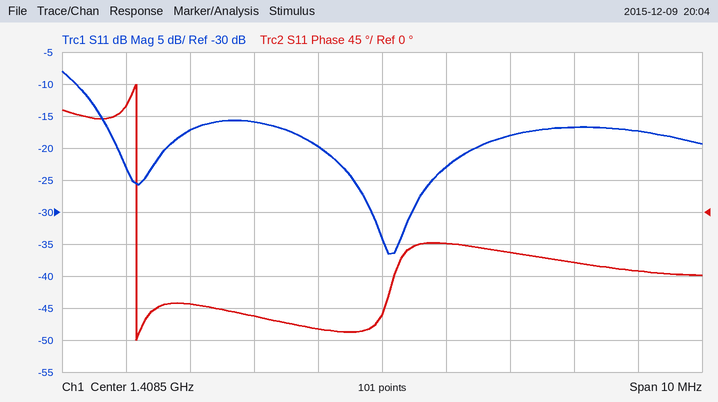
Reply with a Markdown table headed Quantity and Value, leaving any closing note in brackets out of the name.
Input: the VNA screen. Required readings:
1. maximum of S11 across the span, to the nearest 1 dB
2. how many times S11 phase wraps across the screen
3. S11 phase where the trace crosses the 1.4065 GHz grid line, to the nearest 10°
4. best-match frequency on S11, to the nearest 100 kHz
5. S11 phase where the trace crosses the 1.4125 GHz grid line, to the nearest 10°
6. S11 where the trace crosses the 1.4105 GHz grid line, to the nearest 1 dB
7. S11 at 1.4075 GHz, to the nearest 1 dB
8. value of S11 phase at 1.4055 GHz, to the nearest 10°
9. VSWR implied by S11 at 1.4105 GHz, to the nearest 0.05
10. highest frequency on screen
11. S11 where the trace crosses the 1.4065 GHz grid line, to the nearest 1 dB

| Quantity | Value |
|---|---|
| maximum of S11 across the span, to the nearest 1 dB | -8 dB |
| how many times S11 phase wraps across the screen | 1 |
| S11 phase where the trace crosses the 1.4065 GHz grid line, to the nearest 10° | -150° |
| best-match frequency on S11, to the nearest 100 kHz | 1.4086 GHz |
| S11 phase where the trace crosses the 1.4125 GHz grid line, to the nearest 10° | -80° |
| S11 where the trace crosses the 1.4105 GHz grid line, to the nearest 1 dB | -18 dB |
| S11 at 1.4075 GHz, to the nearest 1 dB | -20 dB |
| value of S11 phase at 1.4055 GHz, to the nearest 10° | -130° |
| VSWR implied by S11 at 1.4105 GHz, to the nearest 0.05 | 1.30 |
| highest frequency on screen | 1.4135 GHz |
| S11 where the trace crosses the 1.4065 GHz grid line, to the nearest 1 dB | -16 dB |
